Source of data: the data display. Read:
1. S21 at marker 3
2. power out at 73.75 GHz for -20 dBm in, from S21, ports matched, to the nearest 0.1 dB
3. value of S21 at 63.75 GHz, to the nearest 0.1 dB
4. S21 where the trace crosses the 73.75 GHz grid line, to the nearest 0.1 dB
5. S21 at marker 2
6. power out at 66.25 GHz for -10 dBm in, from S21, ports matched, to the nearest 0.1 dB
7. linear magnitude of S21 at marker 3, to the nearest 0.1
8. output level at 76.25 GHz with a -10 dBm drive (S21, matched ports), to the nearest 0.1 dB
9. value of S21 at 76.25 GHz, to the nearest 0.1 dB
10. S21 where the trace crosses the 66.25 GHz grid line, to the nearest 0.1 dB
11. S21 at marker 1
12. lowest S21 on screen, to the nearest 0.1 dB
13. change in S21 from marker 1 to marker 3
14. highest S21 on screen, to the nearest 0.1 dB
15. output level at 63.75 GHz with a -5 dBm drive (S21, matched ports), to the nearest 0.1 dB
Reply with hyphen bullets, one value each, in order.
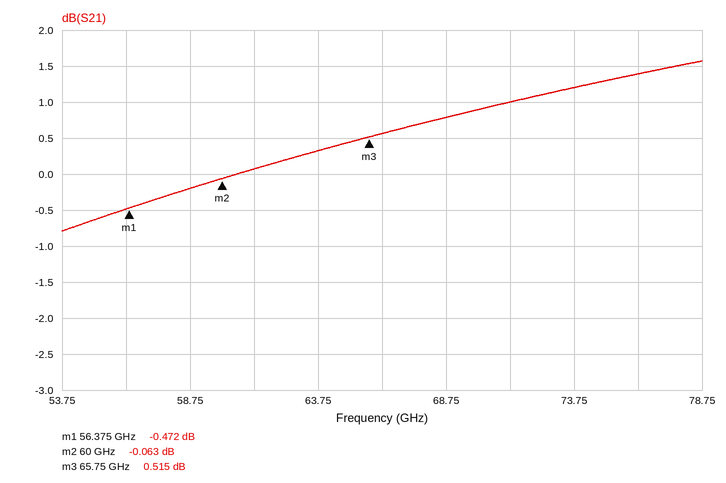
- 0.515 dB
- -18.8 dBm
- 0.3 dB
- 1.2 dB
- -0.063 dB
- -9.4 dBm
- 1.1
- -8.6 dBm
- 1.4 dB
- 0.6 dB
- -0.472 dB
- -0.8 dB
- 0.987 dB
- 1.6 dB
- -4.7 dBm
